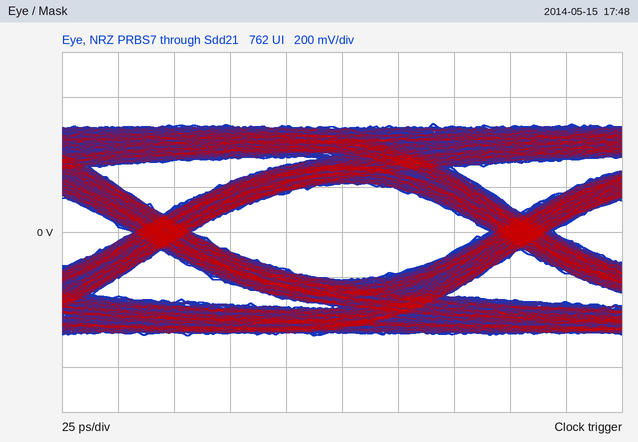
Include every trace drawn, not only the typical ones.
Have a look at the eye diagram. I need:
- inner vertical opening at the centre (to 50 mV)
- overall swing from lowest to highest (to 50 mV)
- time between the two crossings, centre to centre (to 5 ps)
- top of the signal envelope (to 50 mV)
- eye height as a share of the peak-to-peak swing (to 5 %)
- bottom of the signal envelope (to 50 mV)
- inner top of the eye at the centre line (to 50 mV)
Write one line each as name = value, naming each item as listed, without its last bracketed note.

inner vertical opening at the centre = 450 mV
overall swing from lowest to highest = 950 mV
time between the two crossings, centre to centre = 160 ps
top of the signal envelope = 500 mV
eye height as a share of the peak-to-peak swing = 45 %
bottom of the signal envelope = -450 mV
inner top of the eye at the centre line = 200 mV
